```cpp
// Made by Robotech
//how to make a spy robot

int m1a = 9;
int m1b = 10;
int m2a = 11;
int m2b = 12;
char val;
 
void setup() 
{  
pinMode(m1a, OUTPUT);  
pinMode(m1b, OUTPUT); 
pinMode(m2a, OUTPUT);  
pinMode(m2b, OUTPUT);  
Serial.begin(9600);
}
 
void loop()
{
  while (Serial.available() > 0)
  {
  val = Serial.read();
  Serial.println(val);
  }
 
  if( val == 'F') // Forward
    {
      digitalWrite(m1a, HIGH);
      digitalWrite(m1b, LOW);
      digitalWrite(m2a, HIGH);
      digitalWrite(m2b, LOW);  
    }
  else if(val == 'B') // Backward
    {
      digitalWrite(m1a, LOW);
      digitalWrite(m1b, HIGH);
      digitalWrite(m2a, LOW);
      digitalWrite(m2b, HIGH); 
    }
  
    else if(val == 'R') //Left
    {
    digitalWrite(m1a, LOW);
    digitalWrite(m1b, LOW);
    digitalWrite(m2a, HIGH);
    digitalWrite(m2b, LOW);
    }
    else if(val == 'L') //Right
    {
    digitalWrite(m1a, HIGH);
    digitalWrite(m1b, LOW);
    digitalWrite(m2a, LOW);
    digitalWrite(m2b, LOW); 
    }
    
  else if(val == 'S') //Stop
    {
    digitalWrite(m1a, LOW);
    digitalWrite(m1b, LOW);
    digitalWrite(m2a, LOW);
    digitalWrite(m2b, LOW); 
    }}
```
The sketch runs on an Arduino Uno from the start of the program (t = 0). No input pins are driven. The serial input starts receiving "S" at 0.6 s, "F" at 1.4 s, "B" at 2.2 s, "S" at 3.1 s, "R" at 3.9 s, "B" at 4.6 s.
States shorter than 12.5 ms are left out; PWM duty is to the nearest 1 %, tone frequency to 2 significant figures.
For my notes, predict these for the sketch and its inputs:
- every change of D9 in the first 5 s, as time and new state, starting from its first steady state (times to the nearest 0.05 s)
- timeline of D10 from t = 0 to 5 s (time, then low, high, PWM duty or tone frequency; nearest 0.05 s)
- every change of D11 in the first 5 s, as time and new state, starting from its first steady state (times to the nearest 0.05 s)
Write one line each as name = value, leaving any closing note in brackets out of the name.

every change of D9 in the first 5 s, as time and new state, starting from its first steady state = 0 s low; 1.4 s high; 2.2 s low
timeline of D10 from t = 0 to 5 s = 0 s low; 2.2 s high; 3.1 s low; 4.6 s high
every change of D11 in the first 5 s, as time and new state, starting from its first steady state = 0 s low; 1.4 s high; 2.2 s low; 3.9 s high; 4.6 s low
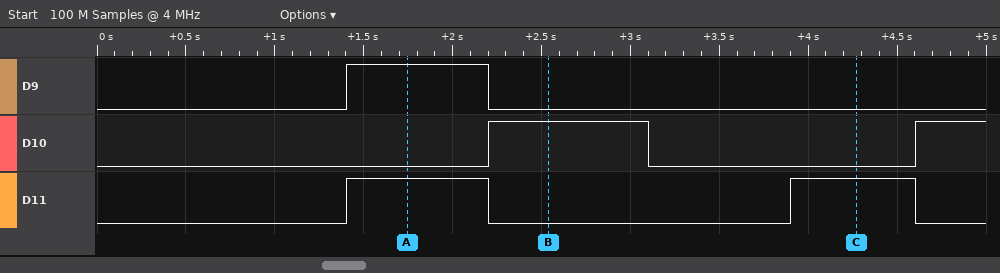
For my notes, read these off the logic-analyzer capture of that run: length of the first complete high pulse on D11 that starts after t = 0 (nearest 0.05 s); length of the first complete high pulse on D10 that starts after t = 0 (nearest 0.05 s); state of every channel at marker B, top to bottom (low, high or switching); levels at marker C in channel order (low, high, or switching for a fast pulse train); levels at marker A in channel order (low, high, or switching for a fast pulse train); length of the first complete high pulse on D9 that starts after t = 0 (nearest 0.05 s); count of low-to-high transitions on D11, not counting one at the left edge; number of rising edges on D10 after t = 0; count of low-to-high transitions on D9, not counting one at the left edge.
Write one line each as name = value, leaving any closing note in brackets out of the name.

length of the first complete high pulse on D11 that starts after t = 0 = 0.80 s
length of the first complete high pulse on D10 that starts after t = 0 = 0.90 s
state of every channel at marker B, top to bottom = D9 low, D10 high, D11 low
levels at marker C in channel order = D9 low, D10 low, D11 high
levels at marker A in channel order = D9 high, D10 low, D11 high
length of the first complete high pulse on D9 that starts after t = 0 = 0.80 s
count of low-to-high transitions on D11, not counting one at the left edge = 2
number of rising edges on D10 after t = 0 = 2
count of low-to-high transitions on D9, not counting one at the left edge = 1
